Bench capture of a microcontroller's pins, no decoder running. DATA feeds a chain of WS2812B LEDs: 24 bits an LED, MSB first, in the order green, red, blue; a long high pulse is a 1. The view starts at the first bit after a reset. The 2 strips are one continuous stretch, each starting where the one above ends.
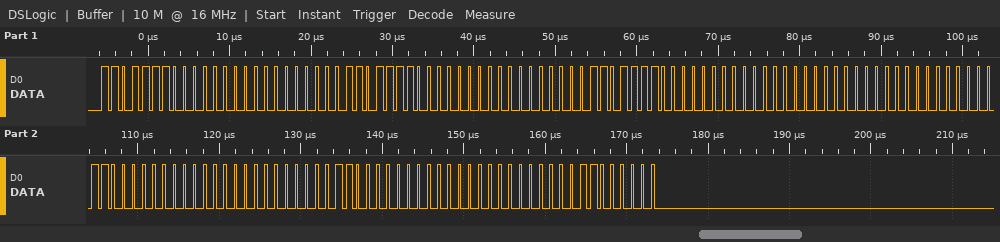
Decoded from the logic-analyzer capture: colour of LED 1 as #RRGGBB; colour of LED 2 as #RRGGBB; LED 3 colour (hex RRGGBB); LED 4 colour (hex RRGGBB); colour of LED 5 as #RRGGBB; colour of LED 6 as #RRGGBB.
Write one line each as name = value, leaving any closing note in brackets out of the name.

colour of LED 1 as #RRGGBB = #00DE00
colour of LED 2 as #RRGGBB = #00DE00
LED 3 colour = #00DE00
LED 4 colour = #0000C0
colour of LED 5 as #RRGGBB = #0000C0
colour of LED 6 as #RRGGBB = #0000C0
